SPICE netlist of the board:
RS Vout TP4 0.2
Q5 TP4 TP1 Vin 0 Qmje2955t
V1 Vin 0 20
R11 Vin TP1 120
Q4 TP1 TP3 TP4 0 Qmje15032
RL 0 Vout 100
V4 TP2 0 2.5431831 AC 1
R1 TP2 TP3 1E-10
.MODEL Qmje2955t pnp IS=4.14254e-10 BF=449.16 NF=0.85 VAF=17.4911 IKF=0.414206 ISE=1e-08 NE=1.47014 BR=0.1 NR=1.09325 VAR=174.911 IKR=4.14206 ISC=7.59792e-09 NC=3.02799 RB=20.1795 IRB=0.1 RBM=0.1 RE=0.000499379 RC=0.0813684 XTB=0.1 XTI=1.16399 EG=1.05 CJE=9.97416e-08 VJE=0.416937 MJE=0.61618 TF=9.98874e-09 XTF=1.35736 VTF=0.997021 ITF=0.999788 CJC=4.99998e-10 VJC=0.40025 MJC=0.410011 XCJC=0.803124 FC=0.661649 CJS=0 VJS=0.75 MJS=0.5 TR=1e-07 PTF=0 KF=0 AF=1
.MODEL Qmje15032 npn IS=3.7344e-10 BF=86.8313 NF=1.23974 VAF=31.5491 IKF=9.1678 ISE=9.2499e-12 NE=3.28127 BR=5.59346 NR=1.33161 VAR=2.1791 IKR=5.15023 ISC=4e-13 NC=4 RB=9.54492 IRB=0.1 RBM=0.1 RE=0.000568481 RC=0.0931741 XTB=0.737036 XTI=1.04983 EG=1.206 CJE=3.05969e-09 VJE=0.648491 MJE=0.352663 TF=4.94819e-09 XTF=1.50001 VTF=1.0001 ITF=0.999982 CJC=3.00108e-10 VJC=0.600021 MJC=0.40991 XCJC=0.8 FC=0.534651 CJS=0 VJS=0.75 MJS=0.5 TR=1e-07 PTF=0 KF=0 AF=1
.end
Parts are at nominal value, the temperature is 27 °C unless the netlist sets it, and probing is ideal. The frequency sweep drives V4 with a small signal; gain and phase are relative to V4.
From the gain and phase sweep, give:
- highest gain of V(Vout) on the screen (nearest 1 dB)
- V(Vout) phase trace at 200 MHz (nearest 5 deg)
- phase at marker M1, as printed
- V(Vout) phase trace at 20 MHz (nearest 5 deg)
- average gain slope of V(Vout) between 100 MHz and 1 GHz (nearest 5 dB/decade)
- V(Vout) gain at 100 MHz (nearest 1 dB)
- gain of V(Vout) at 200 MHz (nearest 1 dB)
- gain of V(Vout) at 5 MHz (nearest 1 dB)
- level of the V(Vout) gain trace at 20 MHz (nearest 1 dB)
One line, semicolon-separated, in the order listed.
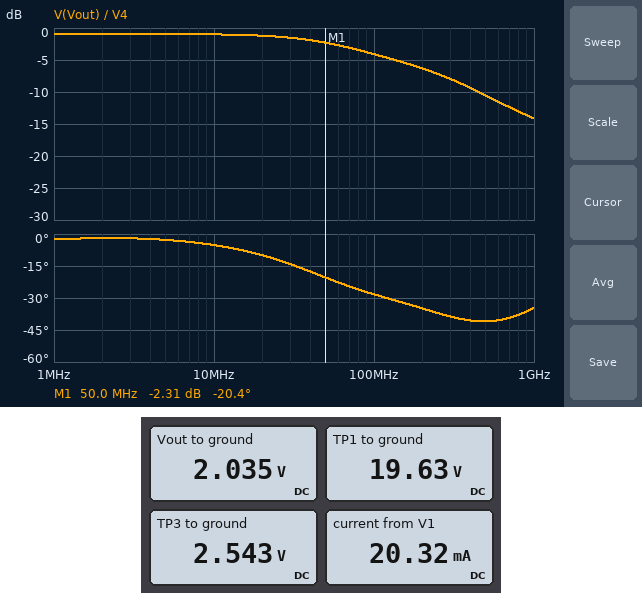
-1 dB; -35 deg; -20.4 deg; -10 deg; -10 dB/decade; -4 dB; -6 dB; -1 dB; -1 dB
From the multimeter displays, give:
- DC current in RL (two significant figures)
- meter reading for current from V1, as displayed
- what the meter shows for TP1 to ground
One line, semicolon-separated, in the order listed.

20 mA; 20.32 mA; 19.63 V
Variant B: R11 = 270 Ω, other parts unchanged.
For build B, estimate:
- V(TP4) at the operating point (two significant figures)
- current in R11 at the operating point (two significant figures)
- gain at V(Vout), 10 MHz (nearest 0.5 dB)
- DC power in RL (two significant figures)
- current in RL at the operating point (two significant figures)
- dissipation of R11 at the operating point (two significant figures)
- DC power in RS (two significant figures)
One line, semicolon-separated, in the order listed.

2.1 V; 1.4 mA; -1.0 dB; 42 mW; 21 mA; 530 µW; 85 µW
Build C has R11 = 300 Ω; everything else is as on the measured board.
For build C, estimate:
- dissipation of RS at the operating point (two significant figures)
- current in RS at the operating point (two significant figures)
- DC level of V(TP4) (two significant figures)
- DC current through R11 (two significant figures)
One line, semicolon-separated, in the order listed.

85 µW; 21 mA; 2.1 V; 1.3 mA
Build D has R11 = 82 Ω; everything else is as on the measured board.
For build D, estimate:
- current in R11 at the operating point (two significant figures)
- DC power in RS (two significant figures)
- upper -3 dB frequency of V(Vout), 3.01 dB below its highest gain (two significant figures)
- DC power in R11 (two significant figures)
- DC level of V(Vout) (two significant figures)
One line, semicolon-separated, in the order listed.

4.5 mA; 82 µW; 70 MHz; 1.7 mW; 2.0 V
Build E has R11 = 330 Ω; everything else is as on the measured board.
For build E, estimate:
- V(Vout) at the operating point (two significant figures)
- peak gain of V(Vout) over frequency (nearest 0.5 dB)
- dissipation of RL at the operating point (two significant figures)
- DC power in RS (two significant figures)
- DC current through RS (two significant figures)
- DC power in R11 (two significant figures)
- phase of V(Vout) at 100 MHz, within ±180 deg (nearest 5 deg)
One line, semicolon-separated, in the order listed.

2.1 V; 0 dB; 43 mW; 85 µW; 21 mA; 430 µW; -25 deg
